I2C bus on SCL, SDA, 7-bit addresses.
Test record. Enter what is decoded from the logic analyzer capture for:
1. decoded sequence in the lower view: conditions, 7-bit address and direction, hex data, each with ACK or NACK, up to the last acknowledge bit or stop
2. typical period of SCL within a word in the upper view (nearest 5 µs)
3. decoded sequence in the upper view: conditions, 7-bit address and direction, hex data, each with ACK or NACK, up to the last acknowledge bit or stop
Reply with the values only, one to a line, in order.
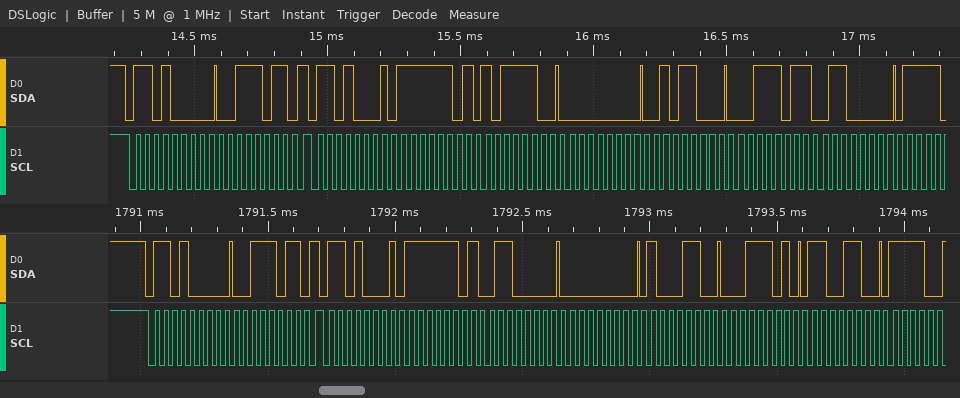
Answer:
start, address 68 write ACK, 3B ACK, repeated start, address 68 read ACK, FD ACK, 60 ACK, 00 ACK, 8C ACK, 3A ACK, CC ACK
35 µs
start, address 68 write ACK, 3B ACK, repeated start, address 68 read ACK, FD ACK, BC ACK, 00 ACK, 58 ACK, 3B ACK, 60 ACK
